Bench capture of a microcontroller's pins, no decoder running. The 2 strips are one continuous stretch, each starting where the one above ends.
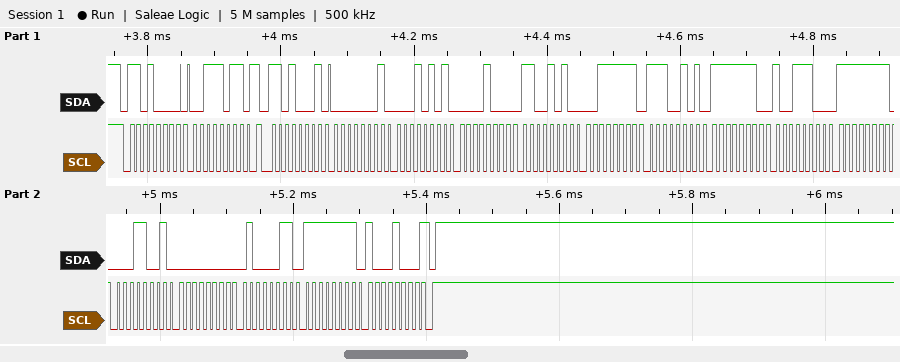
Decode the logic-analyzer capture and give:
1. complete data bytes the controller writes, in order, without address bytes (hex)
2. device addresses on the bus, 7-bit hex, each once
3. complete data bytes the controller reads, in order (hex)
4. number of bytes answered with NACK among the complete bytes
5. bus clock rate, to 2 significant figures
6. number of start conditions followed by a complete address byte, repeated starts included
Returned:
3B
0x68
01 15 08 CA 3F E5 FE 9C FF 19 00 43 FF 88
1
100 kHz
2
